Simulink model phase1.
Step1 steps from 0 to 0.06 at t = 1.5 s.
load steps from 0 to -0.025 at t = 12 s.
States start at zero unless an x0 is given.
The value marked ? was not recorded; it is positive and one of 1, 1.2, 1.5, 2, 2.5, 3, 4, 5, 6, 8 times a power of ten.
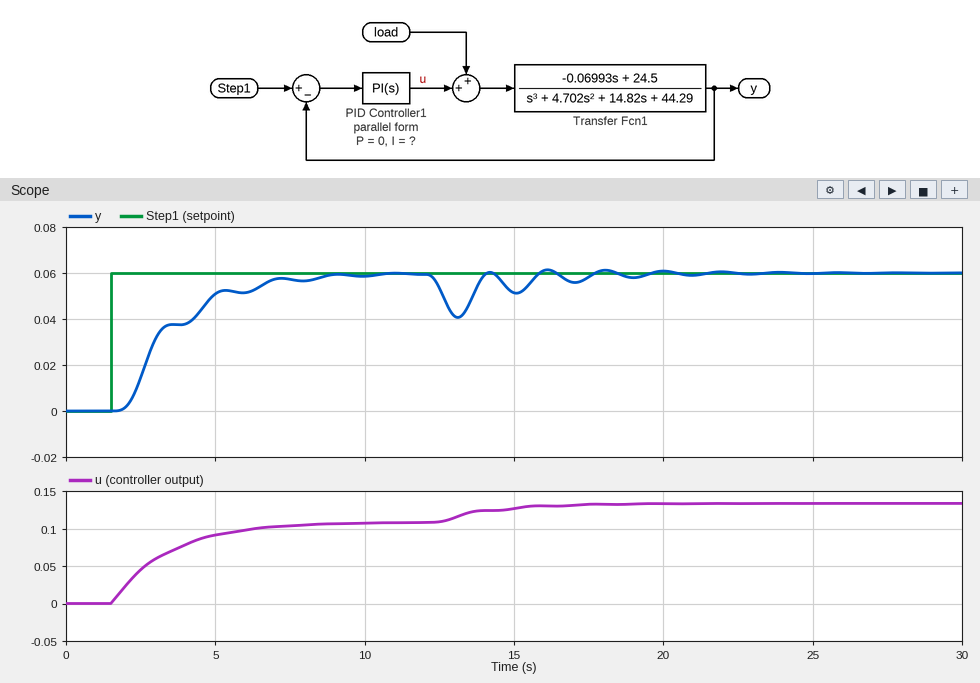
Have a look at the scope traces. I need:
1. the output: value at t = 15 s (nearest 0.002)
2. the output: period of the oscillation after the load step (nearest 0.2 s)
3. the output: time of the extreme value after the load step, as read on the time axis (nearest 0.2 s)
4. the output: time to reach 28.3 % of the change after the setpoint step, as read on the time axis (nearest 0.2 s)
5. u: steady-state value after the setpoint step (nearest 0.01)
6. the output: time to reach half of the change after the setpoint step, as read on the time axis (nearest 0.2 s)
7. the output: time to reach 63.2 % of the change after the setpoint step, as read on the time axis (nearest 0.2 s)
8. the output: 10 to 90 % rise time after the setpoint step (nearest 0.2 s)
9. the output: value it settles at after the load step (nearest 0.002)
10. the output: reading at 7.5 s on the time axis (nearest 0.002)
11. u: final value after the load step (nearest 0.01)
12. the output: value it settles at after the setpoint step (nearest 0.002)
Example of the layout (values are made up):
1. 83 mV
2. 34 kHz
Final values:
1. 0.052
2. 2.0 s
3. 13.2 s
4. 2.6 s
5. 0.11
6. 3.0 s
7. 4.0 s
8. 4.2 s
9. 0.060
10. 0.058
11. 0.13
12. 0.060
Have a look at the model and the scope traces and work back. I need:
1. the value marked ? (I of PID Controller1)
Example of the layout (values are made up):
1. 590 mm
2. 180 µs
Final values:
1. 0.8
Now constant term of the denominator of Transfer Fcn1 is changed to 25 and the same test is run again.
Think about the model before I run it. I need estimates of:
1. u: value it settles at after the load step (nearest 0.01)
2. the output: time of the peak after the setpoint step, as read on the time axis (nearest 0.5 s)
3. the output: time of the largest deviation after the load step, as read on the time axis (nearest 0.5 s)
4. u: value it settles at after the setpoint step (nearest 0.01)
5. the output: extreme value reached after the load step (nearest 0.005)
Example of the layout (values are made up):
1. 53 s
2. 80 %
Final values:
1. 0.09
2. 4.0 s
3. 13.5 s
4. 0.06
5. 0.035
